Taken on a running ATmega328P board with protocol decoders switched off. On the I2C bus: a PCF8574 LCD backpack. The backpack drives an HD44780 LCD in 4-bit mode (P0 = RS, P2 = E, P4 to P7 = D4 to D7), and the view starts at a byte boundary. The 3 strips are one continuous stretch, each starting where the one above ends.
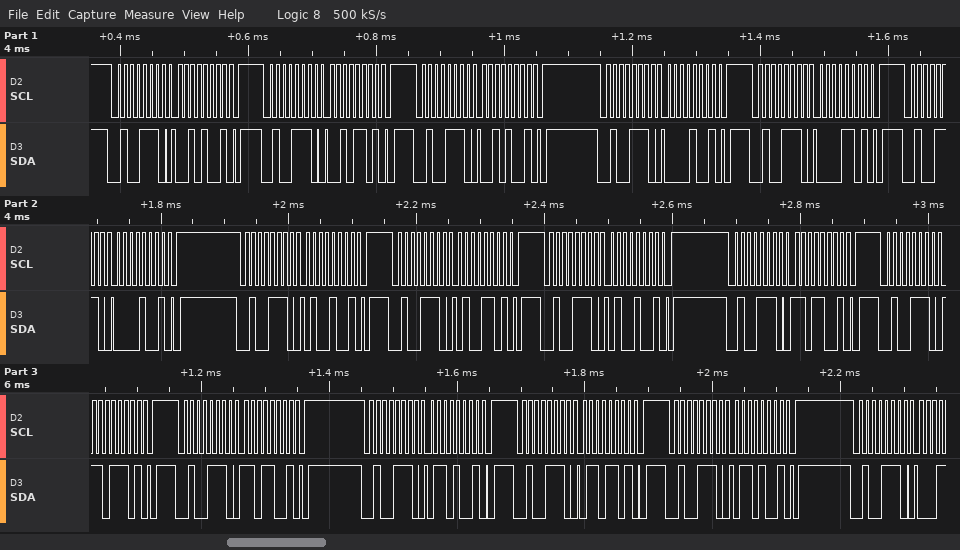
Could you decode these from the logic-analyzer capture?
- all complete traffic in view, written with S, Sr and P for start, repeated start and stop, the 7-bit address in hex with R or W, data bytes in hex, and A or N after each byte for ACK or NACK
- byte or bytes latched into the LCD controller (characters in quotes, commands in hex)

S 27W A 29 A P S 27W A 2D A P S 27W A 29 A P S 27W A 09 A P S 27W A 0D A P S 27W A 09 A P S 27W A 49 A P S 27W A 4D A P S 27W A 49 A P S 27W A D9 A P S 27W A DD A P S 27W A D9 A P S 27W A 69 A P S 27W A 6D A P S 27W A 69 A P S 27W A
' ' 'M'
